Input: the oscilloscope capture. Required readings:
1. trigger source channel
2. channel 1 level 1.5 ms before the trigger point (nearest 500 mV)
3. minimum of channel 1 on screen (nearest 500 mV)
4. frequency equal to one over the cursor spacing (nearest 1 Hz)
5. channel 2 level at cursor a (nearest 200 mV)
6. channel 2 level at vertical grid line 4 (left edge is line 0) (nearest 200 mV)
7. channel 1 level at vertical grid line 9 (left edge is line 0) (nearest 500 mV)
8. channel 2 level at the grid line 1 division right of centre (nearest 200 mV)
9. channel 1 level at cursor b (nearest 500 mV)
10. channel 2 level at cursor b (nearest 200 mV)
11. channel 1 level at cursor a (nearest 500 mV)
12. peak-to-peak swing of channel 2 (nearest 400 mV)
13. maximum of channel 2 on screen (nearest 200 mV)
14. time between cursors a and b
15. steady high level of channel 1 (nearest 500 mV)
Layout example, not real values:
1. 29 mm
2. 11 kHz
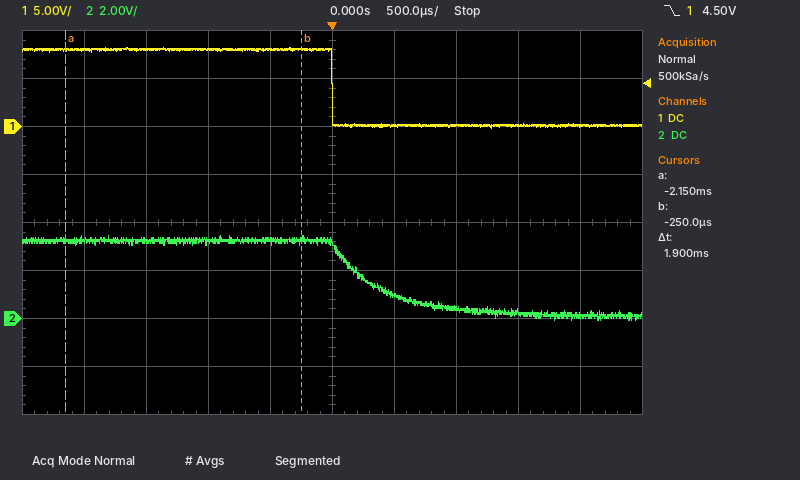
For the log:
1. channel 1
2. 8.0 V
3. 0.0 V
4. 526 Hz
5. 3.2 V
6. 3.2 V
7. 0.0 V
8. 1.0 V
9. 8.0 V
10. 3.2 V
11. 8.0 V
12. 3.6 V
13. 3.4 V
14. 1.9 ms
15. 8.0 V
